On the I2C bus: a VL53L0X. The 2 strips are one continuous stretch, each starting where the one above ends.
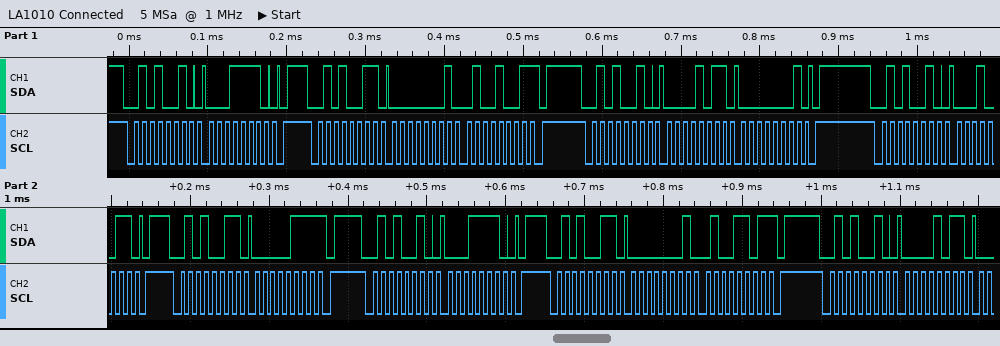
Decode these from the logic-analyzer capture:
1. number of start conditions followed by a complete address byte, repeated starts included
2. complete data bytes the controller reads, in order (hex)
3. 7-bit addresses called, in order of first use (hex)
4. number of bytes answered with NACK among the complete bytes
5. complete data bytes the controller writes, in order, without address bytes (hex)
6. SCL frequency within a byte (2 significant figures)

8
01 49 07 01 4D
0x29
3
1E 0B 01 13 1E 0B
100 kHz
